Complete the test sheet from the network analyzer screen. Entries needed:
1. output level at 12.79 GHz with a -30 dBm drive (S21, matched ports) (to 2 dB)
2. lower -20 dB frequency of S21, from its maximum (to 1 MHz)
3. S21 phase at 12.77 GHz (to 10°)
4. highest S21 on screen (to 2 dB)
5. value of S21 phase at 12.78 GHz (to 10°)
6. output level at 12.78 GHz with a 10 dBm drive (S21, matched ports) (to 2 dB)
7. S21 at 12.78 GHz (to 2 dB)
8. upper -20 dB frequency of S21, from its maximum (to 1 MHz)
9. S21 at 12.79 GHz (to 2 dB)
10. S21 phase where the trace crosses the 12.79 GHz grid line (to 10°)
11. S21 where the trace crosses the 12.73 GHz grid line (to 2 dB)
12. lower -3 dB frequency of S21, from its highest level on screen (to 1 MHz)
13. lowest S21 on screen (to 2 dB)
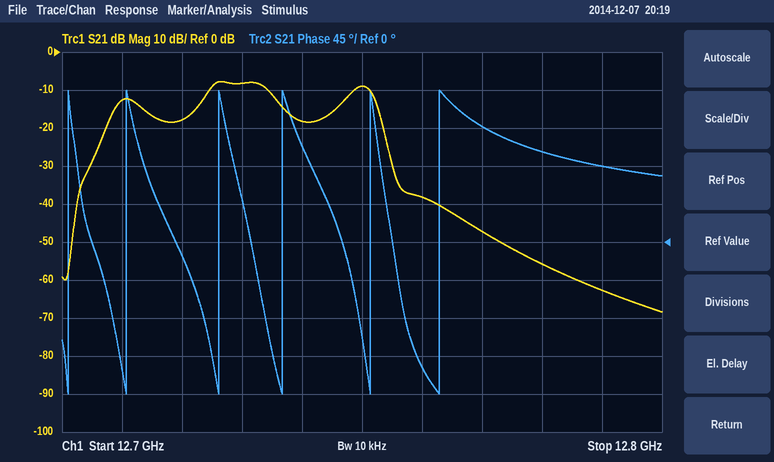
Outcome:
-92 dBm
12.705 GHz
140°
-8 dB
110°
-46 dBm
-56 dB
12.755 GHz
-62 dB
90°
-8 dB
12.724 GHz
-68 dB
